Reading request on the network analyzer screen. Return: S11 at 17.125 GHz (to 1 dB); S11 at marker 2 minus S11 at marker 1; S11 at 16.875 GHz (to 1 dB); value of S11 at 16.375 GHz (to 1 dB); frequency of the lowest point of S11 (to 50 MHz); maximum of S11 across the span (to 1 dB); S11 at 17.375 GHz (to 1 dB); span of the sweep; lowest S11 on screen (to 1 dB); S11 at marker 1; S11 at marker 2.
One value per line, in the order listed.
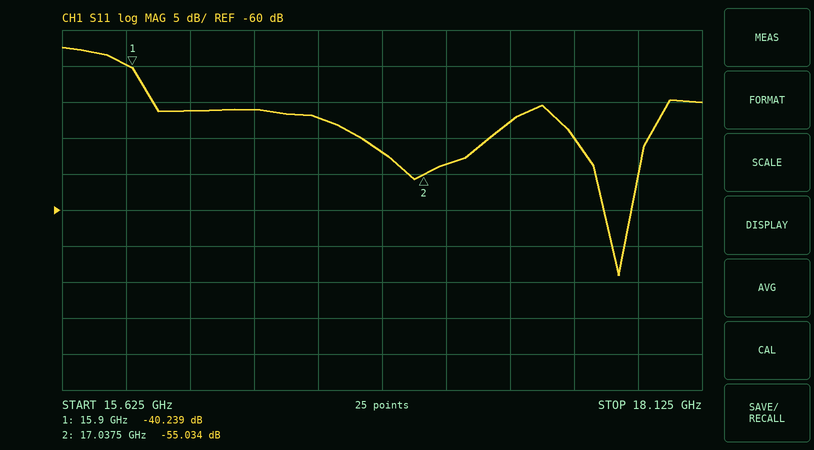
-54 dB
-14.795 dB
-52 dB
-46 dB
17.80 GHz
-37 dB
-48 dB
2.5 GHz
-69 dB
-40.239 dB
-55.034 dB
